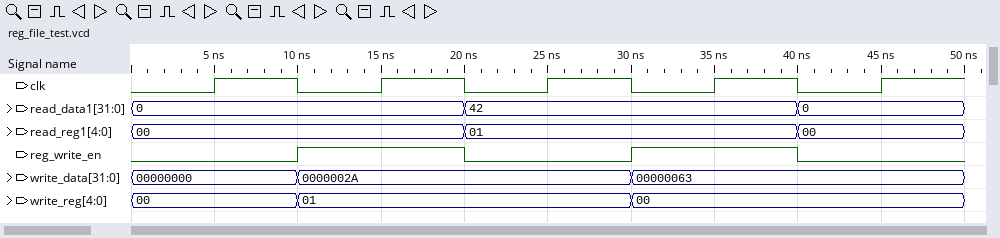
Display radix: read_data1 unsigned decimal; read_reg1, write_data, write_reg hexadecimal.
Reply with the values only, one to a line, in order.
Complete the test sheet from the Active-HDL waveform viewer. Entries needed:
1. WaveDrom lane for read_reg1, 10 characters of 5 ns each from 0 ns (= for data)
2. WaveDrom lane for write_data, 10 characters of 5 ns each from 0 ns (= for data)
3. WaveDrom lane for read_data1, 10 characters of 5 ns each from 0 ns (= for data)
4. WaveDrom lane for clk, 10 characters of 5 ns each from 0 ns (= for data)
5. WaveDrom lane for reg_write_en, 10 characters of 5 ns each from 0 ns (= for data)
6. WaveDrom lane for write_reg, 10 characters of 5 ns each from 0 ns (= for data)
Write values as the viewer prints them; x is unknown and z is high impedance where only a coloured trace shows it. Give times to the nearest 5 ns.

{name: 'read_reg1', wave: '=...=...=.', data: '00 01 00'}
{name: 'write_data', wave: '=.=...=...', data: '00000000 0000002A 00000063'}
{name: 'read_data1', wave: '=...=...=.', data: '0 42 0'}
{name: 'clk', wave: '0101010101'}
{name: 'reg_write_en', wave: '0.1.0.1.0.'}
{name: 'write_reg', wave: '=.=...=...', data: '00 01 00'}
